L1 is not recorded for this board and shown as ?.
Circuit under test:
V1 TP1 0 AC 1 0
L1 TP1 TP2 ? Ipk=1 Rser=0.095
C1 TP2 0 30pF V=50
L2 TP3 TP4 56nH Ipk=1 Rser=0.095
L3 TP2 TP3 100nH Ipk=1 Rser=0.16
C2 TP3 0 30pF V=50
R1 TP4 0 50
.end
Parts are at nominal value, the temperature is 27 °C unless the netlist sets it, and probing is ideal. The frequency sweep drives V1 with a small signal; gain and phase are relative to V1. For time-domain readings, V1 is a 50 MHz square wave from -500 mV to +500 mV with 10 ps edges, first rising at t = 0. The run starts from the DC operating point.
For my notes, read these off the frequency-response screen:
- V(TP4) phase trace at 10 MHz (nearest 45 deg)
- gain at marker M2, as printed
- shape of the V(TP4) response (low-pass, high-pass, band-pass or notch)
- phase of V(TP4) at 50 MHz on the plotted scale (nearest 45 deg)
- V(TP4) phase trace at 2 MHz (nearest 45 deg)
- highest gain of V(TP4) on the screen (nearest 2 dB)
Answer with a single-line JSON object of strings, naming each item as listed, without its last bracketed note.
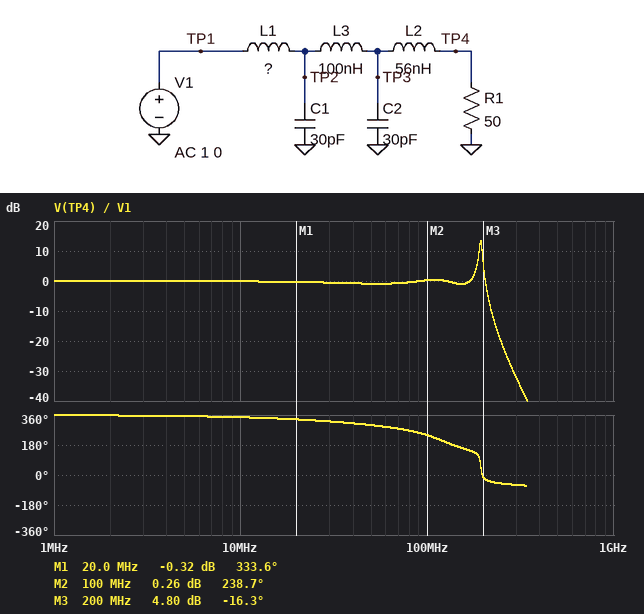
{"V(TP4) phase trace at 10 MHz": "360 deg", "gain at marker M2, as printed": "0.26 dB", "shape of the V(TP4) response": "band-pass", "phase of V(TP4) at 50 MHz on the plotted scale": "315 deg", "V(TP4) phase trace at 2 MHz": "360 deg", "highest gain of V(TP4) on the screen": "14 dB"}
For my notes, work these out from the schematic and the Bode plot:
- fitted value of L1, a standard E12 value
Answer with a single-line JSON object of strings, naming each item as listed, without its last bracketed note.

{"fitted value of L1, a standard E12 value": "33 nH"}
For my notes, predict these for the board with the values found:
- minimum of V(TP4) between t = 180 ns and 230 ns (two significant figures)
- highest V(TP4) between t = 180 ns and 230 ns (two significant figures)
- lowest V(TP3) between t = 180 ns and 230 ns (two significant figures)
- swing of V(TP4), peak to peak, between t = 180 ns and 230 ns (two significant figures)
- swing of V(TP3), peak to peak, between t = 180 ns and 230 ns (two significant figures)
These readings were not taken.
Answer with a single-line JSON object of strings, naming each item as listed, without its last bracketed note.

{"minimum of V(TP4) between t = 180 ns and 230 ns": "-580 mV", "highest V(TP4) between t = 180 ns and 230 ns": "580 mV", "lowest V(TP3) between t = 180 ns and 230 ns": "-720 mV", "swing of V(TP4), peak to peak, between t = 180 ns and 230 ns": "1.2 V", "swing of V(TP3), peak to peak, between t = 180 ns and 230 ns": "1.4 V"}
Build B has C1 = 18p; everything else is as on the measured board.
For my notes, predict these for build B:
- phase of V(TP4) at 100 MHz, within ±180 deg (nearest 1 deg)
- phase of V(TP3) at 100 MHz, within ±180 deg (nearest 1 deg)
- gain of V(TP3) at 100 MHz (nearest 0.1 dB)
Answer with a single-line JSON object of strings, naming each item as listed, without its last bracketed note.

{"phase of V(TP4) at 100 MHz, within ±180 deg": "-118 deg", "phase of V(TP3) at 100 MHz, within ±180 deg": "-83 deg", "gain of V(TP3) at 100 MHz": "0.6 dB"}
